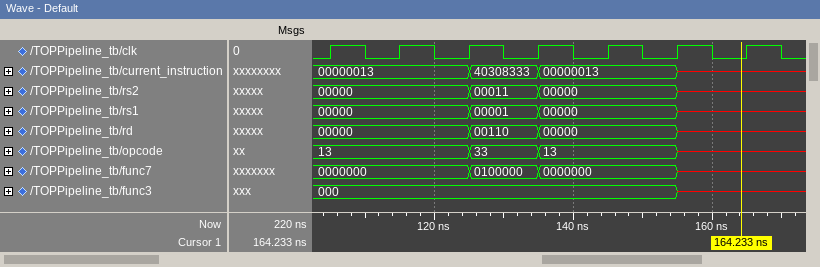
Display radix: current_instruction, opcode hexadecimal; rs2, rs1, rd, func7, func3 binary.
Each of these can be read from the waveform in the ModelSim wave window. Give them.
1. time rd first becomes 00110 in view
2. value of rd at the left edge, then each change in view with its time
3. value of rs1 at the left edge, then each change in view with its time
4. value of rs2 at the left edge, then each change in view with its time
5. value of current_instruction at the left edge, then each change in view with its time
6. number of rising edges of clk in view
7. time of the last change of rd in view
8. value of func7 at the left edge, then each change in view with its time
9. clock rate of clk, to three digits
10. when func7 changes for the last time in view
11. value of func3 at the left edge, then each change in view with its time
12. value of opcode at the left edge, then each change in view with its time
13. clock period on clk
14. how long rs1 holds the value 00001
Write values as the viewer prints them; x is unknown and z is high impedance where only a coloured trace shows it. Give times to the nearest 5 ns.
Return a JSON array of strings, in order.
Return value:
["125 ns", "00000, 00110 at 125 ns, 00000 at 135 ns, x at 155 ns", "00000, 00001 at 125 ns, 00000 at 135 ns, x at 155 ns", "00000, 00011 at 125 ns, 00000 at 135 ns, x at 155 ns", "00000013, 40308333 at 125 ns, 00000013 at 135 ns, x at 155 ns", "7", "155 ns", "0000000, 0100000 at 125 ns, 0000000 at 135 ns, x at 155 ns", "100 MHz", "155 ns", "000, x at 155 ns", "13, 33 at 125 ns, 13 at 135 ns, x at 155 ns", "10 ns", "10 ns"]
